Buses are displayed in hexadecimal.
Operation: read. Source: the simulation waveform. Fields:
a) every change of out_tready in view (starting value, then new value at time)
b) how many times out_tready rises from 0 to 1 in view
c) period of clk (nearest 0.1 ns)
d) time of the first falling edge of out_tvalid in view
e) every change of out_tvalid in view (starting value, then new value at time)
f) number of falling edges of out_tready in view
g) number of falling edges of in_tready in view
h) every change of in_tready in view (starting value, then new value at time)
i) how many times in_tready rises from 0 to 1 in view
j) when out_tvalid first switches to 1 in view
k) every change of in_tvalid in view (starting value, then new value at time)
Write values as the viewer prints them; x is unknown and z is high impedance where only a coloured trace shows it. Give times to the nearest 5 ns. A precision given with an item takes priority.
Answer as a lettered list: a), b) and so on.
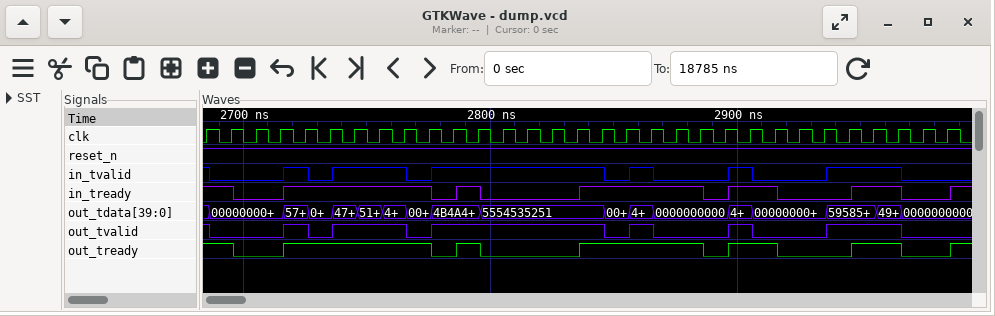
a) 1, 0 at 2695 ns, 1 at 2715 ns, 0 at 2775 ns, 1 at 2785 ns, 0 at 2795 ns, 1 at 2835 ns, 0 at 2885 ns, 1 at 2895 ns, 0 at 2915 ns, 1 at 2945 ns, 0 at 2965 ns, 1 at 2985 ns
b) 6
c) 10 ns
d) 2685 ns
e) 1, 0 at 2685 ns, 1 at 2715 ns, 0 at 2725 ns, 1 at 2735 ns, 0 at 2765 ns, 1 at 2775 ns, 0 at 2845 ns, 1 at 2855 ns, 0 at 2865 ns, 1 at 2895 ns, 0 at 2905 ns, 1 at 2935 ns, 0 at 2965 ns
f) 6
g) 6
h) 1, 0 at 2695 ns, 1 at 2715 ns, 0 at 2775 ns, 1 at 2785 ns, 0 at 2795 ns, 1 at 2835 ns, 0 at 2885 ns, 1 at 2895 ns, 0 at 2915 ns, 1 at 2945 ns, 0 at 2965 ns, 1 at 2985 ns
i) 6
j) 2715 ns
k) 1, 0 at 2685 ns, 1 at 2715 ns, 0 at 2725 ns, 1 at 2735 ns, 0 at 2765 ns, 1 at 2775 ns, 0 at 2845 ns, 1 at 2855 ns, 0 at 2865 ns, 1 at 2895 ns, 0 at 2905 ns, 1 at 2935 ns, 0 at 2965 ns
